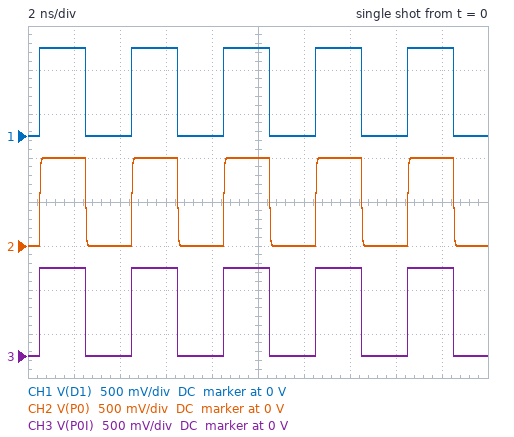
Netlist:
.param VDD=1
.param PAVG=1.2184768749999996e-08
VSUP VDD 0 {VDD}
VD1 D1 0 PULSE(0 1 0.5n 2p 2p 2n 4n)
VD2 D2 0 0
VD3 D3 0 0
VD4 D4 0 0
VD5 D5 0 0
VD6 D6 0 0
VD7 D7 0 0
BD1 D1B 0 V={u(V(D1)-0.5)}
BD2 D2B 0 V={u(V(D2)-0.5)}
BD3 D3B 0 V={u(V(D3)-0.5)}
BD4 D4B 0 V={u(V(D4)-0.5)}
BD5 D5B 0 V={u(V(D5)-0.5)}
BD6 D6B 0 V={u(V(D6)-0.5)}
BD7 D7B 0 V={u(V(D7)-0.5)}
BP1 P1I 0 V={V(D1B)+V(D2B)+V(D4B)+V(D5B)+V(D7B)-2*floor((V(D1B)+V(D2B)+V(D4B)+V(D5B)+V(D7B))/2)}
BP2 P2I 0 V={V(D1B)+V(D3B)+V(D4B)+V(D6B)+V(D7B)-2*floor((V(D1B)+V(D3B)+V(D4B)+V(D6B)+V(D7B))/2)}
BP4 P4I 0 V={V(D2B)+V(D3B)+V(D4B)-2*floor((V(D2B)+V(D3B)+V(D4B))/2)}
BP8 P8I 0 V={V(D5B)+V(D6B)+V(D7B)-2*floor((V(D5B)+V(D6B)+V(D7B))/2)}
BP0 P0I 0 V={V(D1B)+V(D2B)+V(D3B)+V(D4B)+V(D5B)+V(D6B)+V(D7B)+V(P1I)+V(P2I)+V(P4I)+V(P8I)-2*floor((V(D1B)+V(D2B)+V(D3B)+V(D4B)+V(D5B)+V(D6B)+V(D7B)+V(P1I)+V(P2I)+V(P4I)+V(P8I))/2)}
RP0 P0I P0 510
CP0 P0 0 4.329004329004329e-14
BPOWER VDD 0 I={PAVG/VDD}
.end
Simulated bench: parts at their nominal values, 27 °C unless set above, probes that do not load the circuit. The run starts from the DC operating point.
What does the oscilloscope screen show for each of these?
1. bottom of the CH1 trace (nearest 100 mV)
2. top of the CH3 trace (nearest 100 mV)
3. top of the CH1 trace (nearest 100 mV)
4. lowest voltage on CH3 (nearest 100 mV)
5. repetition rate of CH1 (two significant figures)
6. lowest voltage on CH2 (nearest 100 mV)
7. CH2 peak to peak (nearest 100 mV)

0 V
1.0 V
1.0 V
0 V
250 MHz
0 V
1.0 V
